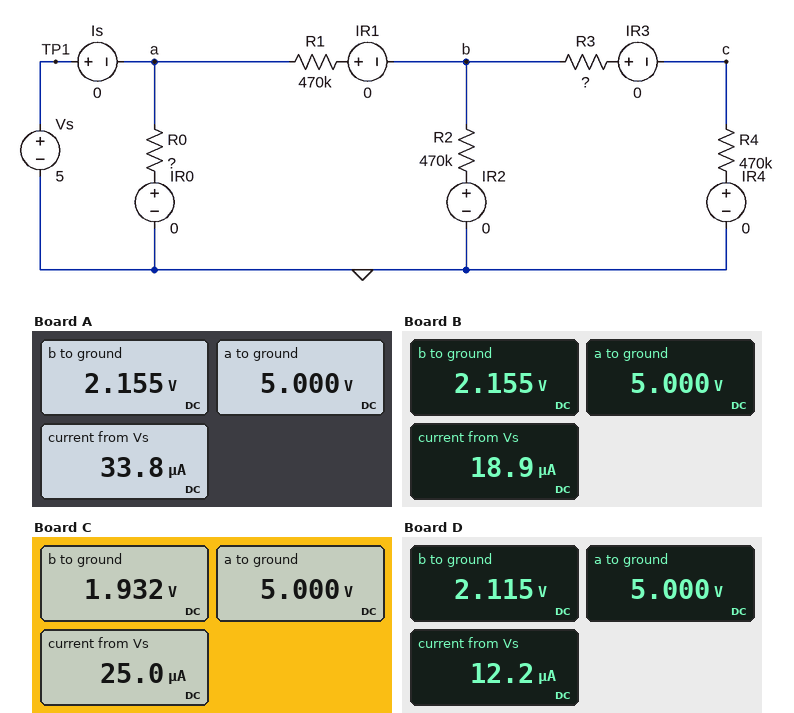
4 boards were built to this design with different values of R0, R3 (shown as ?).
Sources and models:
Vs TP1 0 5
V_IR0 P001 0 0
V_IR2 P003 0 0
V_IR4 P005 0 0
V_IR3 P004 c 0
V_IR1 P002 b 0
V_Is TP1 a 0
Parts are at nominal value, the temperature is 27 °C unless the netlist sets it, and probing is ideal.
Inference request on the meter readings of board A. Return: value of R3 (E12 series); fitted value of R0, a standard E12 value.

1 MΩ
180 kΩ
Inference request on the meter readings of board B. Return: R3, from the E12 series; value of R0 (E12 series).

1 MΩ
390 kΩ
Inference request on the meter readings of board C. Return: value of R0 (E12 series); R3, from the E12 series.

270 kΩ
330 kΩ
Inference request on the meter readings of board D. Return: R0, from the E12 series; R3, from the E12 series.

820 kΩ
820 kΩ
